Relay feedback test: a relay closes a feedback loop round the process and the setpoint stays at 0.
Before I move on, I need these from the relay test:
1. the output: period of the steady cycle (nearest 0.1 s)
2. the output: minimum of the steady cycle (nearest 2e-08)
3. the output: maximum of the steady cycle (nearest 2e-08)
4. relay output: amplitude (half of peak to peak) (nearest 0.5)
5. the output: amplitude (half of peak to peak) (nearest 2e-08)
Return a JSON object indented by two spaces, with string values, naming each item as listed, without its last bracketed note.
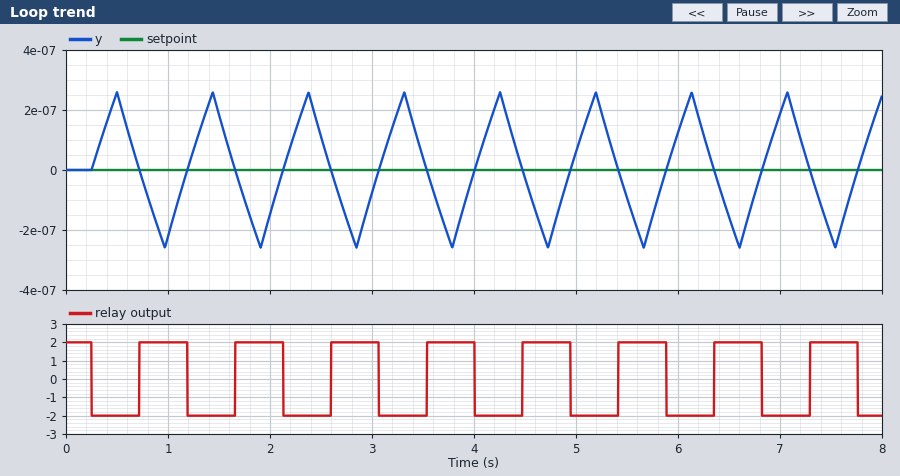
{
  "the output: period of the steady cycle": "0.9 s",
  "the output: minimum of the steady cycle": "-0.00000026",
  "the output: maximum of the steady cycle": "0.00000026",
  "relay output: amplitude (half of peak to peak)": "2.0",
  "the output: amplitude (half of peak to peak)": "0.00000026"
}
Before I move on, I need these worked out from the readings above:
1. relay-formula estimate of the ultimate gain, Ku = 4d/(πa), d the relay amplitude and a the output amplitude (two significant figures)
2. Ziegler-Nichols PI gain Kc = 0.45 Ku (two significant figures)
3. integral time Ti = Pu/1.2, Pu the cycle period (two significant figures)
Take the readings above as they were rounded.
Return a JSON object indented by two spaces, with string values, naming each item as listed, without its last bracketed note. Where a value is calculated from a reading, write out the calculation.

{
  "relay-formula estimate of the ultimate gain, Ku = 4d/(πa), d the relay amplitude and a the output amplitude": "4 × 2 / (π × 2.6e-07) = 9800000",
  "Ziegler-Nichols PI gain Kc = 0.45 Ku": "0.45 × 9.8e+06 = 4400000",
  "integral time Ti = Pu/1.2, Pu the cycle period": "0.9 / 1.2 = 0.75 s"
}
